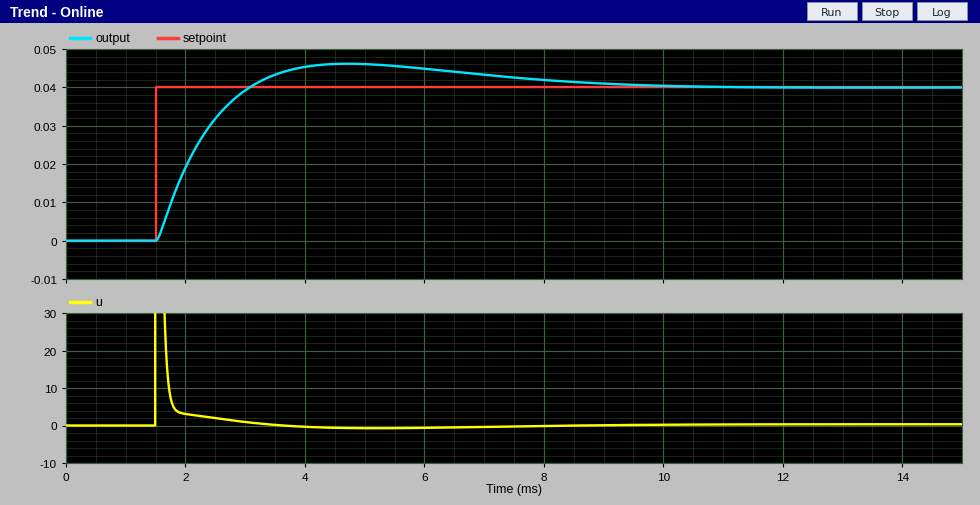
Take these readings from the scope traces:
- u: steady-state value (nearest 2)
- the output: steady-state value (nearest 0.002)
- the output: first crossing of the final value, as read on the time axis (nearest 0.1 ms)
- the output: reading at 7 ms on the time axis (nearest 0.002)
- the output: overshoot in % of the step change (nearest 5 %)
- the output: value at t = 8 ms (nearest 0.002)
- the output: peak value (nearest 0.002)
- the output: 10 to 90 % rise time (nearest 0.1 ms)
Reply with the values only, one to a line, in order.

0
0.040
3.1 ms
0.044
15 %
0.042
0.046
1.1 ms
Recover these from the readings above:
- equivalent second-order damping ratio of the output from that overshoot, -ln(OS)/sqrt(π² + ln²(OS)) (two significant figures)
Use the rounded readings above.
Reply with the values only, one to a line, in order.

0.52
